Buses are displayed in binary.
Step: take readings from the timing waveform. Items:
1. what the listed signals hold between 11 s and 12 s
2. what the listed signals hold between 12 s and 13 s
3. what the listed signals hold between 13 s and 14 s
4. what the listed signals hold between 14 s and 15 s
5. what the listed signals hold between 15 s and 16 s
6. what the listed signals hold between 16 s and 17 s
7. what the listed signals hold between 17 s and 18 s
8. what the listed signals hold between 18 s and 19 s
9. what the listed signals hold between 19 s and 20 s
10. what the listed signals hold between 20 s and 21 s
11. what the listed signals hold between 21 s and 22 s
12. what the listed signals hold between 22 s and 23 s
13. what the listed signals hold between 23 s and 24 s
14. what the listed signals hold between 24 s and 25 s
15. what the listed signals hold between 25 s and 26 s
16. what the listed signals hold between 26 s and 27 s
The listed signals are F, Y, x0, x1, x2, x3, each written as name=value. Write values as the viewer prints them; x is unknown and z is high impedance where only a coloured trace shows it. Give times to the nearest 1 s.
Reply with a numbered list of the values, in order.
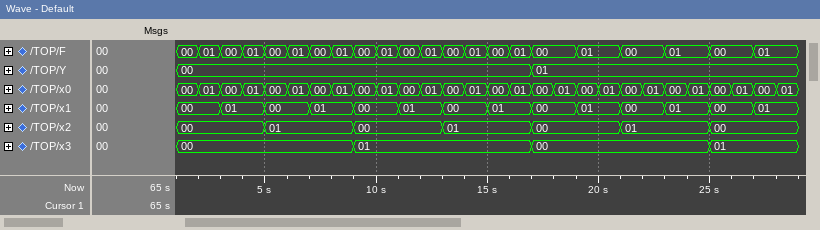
1. F=00, Y=00, x0=00, x1=01, x2=00, x3=01
2. F=01, Y=00, x0=01, x1=01, x2=00, x3=01
3. F=00, Y=00, x0=00, x1=00, x2=01, x3=01
4. F=01, Y=00, x0=01, x1=00, x2=01, x3=01
5. F=00, Y=00, x0=00, x1=01, x2=01, x3=01
6. F=01, Y=00, x0=01, x1=01, x2=01, x3=01
7. F=00, Y=01, x0=00, x1=00, x2=00, x3=00
8. F=00, Y=01, x0=01, x1=00, x2=00, x3=00
9. F=01, Y=01, x0=00, x1=01, x2=00, x3=00
10. F=01, Y=01, x0=01, x1=01, x2=00, x3=00
11. F=00, Y=01, x0=00, x1=00, x2=01, x3=00
12. F=00, Y=01, x0=01, x1=00, x2=01, x3=00
13. F=01, Y=01, x0=00, x1=01, x2=01, x3=00
14. F=01, Y=01, x0=01, x1=01, x2=01, x3=00
15. F=00, Y=01, x0=00, x1=00, x2=00, x3=01
16. F=00, Y=01, x0=01, x1=00, x2=00, x3=01
